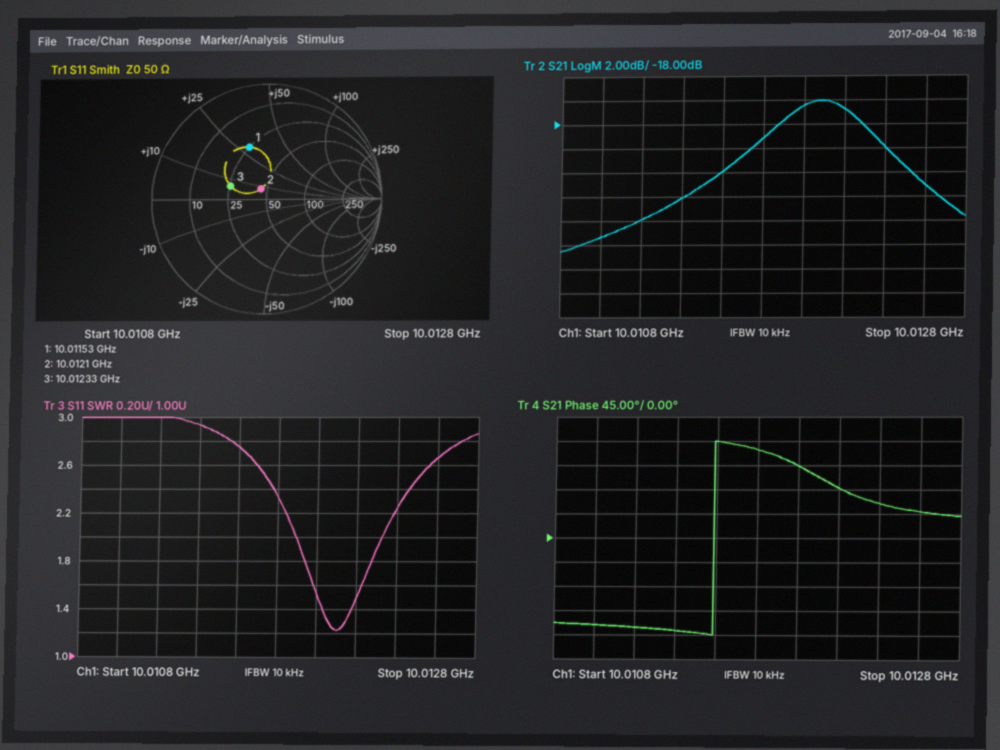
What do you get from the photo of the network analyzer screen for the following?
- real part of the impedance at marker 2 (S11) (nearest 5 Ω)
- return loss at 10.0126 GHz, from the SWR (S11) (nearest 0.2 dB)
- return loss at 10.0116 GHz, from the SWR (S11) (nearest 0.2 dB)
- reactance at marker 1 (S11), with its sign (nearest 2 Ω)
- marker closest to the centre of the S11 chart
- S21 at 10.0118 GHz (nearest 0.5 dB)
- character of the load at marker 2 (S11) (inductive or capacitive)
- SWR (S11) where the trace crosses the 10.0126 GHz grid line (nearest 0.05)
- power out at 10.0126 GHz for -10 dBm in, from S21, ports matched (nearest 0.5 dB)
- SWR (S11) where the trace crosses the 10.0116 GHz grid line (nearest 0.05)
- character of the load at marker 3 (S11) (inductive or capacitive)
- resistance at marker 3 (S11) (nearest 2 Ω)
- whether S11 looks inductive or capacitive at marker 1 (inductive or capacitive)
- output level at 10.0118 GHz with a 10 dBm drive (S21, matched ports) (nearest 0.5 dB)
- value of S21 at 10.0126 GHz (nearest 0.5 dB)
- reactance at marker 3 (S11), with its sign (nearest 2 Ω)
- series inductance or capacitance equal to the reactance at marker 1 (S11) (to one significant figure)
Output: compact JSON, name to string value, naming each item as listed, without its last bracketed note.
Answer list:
{"real part of the impedance at marker 2 (S11)": "45 Ω", "return loss at 10.0126 GHz, from the SWR (S11)": "6.8 dB", "return loss at 10.0116 GHz, from the SWR (S11)": "6.6 dB", "reactance at marker 1 (S11), with its sign": "+30 Ω", "marker closest to the centre of the S11 chart": "marker 2", "S21 at 10.0118 GHz": "-19.0 dB", "character of the load at marker 2 (S11)": "inductive", "SWR (S11) where the trace crosses the 10.0126 GHz grid line": "2.65", "power out at 10.0126 GHz for -10 dBm in, from S21, ports matched": "-33.0 dBm", "SWR (S11) where the trace crosses the 10.0116 GHz grid line": "2.75", "character of the load at marker 3 (S11)": "inductive", "resistance at marker 3 (S11)": "26 Ω", "whether S11 looks inductive or capacitive at marker 1": "inductive", "output level at 10.0118 GHz with a 10 dBm drive (S21, matched ports)": "-9.0 dBm", "value of S21 at 10.0126 GHz": "-23.0 dB", "reactance at marker 3 (S11), with its sign": "+6 Ω", "series inductance or capacitance equal to the reactance at marker 1 (S11)": "500 pH"}
